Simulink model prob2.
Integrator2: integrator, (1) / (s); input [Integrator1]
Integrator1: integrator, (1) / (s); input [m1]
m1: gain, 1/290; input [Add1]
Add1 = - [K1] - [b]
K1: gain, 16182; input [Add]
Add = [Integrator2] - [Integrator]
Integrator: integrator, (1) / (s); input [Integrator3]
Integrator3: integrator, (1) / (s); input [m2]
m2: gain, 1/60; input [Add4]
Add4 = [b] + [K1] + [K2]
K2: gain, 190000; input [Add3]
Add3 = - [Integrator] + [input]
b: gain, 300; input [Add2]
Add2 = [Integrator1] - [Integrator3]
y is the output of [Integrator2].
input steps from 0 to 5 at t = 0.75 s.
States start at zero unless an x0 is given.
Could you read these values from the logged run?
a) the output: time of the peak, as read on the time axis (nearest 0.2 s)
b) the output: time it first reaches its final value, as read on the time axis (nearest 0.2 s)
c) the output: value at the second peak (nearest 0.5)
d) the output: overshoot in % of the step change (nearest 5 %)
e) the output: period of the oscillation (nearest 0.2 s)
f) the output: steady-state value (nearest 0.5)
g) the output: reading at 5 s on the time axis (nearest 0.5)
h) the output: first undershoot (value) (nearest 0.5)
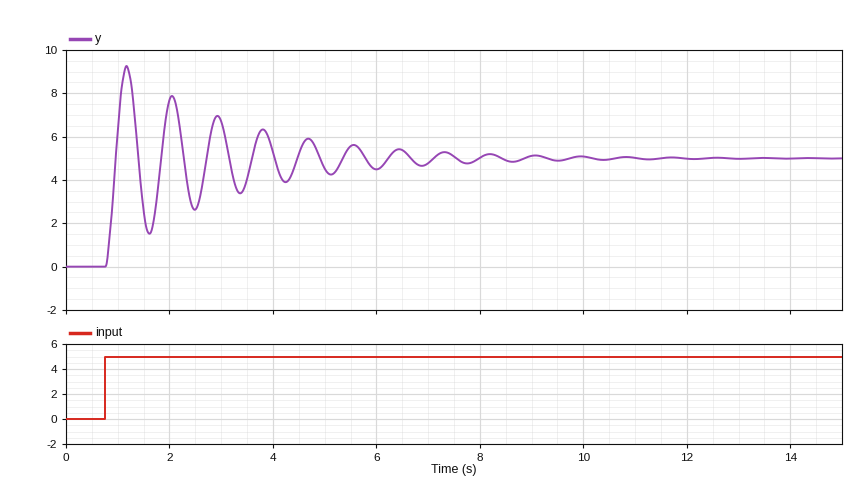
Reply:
1.2 s
1.0 s
8.0
85 %
0.8 s
5.0
4.5
1.5
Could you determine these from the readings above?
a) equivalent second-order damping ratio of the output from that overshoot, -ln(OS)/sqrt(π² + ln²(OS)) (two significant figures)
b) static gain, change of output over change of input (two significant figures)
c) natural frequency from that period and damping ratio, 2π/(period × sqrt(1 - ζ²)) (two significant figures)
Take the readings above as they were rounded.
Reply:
0.052
1.0
7.9 rad/s
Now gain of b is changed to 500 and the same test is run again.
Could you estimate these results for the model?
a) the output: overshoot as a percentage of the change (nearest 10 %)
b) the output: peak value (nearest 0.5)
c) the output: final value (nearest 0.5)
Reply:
80 %
9.0
5.0
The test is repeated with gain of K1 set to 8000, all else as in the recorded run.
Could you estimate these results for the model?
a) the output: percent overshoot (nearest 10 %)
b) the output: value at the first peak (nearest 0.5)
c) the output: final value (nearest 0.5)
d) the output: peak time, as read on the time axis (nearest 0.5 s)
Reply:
80 %
9.0
5.0
1.5 s
